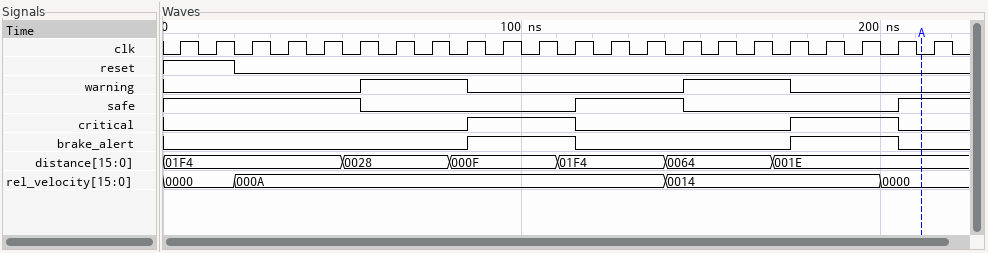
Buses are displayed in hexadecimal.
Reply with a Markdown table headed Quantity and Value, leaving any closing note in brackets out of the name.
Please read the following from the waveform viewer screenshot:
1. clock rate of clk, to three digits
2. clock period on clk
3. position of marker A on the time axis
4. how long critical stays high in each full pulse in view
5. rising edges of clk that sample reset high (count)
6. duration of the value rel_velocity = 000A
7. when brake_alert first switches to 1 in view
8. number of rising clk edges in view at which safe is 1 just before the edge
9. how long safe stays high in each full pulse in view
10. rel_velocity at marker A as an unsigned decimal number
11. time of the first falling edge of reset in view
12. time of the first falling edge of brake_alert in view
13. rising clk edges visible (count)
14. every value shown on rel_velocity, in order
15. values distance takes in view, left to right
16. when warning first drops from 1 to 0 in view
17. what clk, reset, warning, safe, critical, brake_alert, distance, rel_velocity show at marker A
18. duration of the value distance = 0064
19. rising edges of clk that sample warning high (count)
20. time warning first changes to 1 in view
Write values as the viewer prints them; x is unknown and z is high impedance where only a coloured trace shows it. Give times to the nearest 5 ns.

| Quantity | Value |
|---|---|
| clock rate of clk, to three digits | 100 MHz |
| clock period on clk | 10 ns |
| position of marker A on the time axis | 210 ns |
| how long critical stays high in each full pulse in view | 30 ns, 30 ns |
| rising edges of clk that sample reset high | 2 |
| duration of the value rel_velocity = 000A | 120 ns |
| when brake_alert first switches to 1 in view | 85 ns |
| number of rising clk edges in view at which safe is 1 just before the edge | 10 |
| how long safe stays high in each full pulse in view | 30 ns |
| rel_velocity at marker A as an unsigned decimal number | 0 |
| time of the first falling edge of reset in view | 20 ns |
| time of the first falling edge of brake_alert in view | 115 ns |
| rising clk edges visible | 22 |
| every value shown on rel_velocity, in order | 0000, 000A, 0014, 0000 |
| values distance takes in view, left to right | 01F4, 0028, 000F, 01F4, 0064, 001E |
| when warning first drops from 1 to 0 in view | 85 ns |
| what clk, reset, warning, safe, critical, brake_alert, distance, rel_velocity show at marker A | clk=0, reset=0, warning=0, safe=1, critical=0, brake_alert=0, distance=001E, rel_velocity=0000 |
| duration of the value distance = 0064 | 30 ns |
| rising edges of clk that sample warning high | 6 |
| time warning first changes to 1 in view | 55 ns |
